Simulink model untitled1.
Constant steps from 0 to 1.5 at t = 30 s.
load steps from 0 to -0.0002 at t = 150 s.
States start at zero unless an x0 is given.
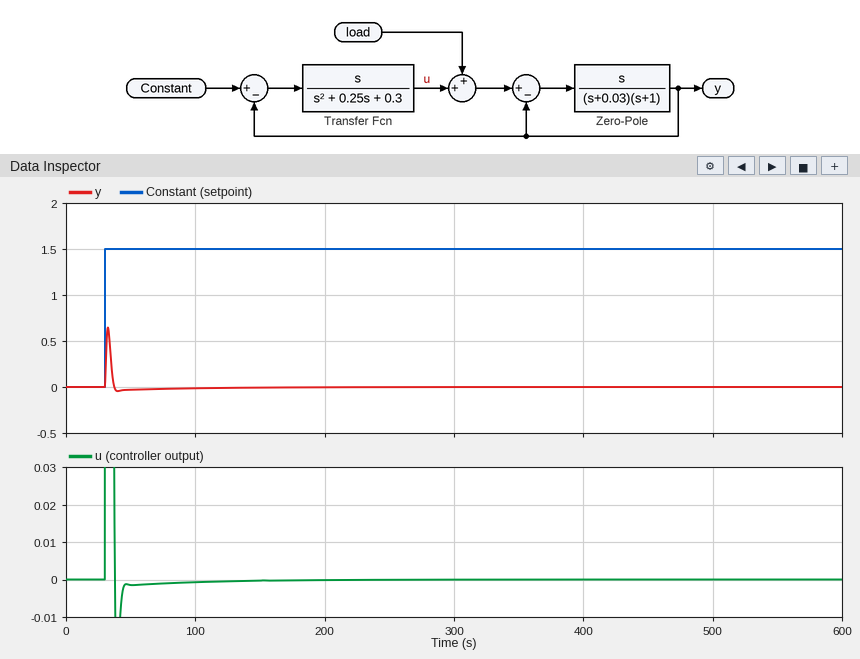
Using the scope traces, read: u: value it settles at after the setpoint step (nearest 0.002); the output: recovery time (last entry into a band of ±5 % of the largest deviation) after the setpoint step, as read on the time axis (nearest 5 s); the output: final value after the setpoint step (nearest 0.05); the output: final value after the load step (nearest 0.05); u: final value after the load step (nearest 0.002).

0.000
45 s
0.00
0.00
0.000
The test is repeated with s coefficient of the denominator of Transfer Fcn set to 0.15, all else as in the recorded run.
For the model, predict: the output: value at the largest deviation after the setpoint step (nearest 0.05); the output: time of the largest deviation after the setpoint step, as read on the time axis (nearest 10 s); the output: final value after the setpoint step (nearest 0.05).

0.70
30 s
0.00
